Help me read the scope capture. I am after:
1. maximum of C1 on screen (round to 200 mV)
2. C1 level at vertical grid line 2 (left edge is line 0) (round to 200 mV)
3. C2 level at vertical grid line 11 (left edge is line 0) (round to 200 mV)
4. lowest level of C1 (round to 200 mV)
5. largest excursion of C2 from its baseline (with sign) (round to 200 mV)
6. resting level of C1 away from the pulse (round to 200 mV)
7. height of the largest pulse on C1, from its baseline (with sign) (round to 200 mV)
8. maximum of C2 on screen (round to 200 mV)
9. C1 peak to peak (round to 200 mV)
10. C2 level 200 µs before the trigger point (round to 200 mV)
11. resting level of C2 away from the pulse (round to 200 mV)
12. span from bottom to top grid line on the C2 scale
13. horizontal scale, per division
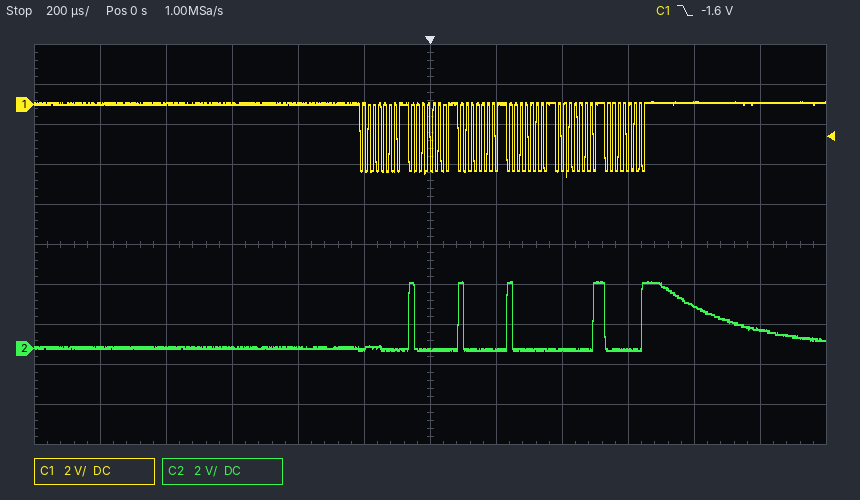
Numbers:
200 mV
0.0 V
1.0 V
-3.6 V
+3.4 V
0.0 V
-3.6 V
3.4 V
3.8 V
0.0 V
0.0 V
20 V
200 µs
